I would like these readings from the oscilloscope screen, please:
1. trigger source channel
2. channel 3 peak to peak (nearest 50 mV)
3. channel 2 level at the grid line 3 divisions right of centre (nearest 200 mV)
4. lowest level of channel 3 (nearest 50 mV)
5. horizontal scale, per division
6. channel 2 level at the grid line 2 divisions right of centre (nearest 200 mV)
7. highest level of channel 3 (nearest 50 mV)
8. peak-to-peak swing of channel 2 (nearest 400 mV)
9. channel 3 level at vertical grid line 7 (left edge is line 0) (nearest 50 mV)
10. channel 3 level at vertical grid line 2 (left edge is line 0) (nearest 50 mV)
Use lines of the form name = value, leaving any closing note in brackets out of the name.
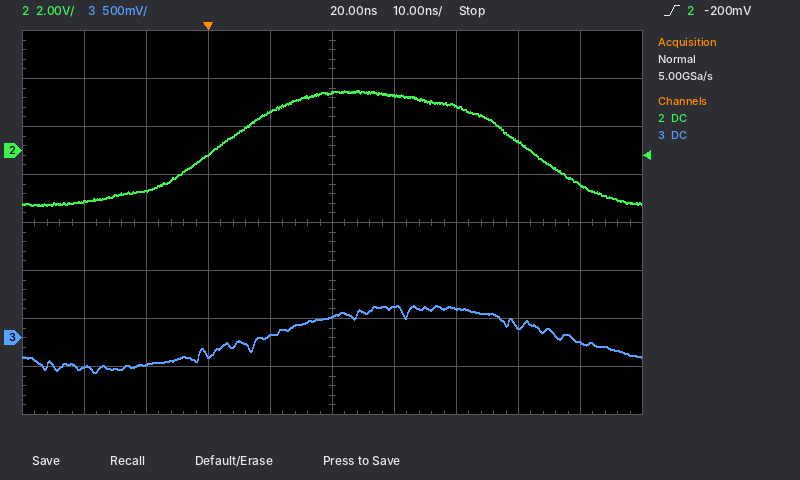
trigger source channel = channel 2
channel 3 peak to peak = 700 mV
channel 2 level at the grid line 3 divisions right of centre = 400 mV
lowest level of channel 3 = -350 mV
horizontal scale, per division = 10 ns
channel 2 level at the grid line 2 divisions right of centre = 1.8 V
highest level of channel 3 = 350 mV
peak-to-peak swing of channel 2 = 4.8 V
channel 3 level at vertical grid line 7 (left edge is line 0) = 300 mV
channel 3 level at vertical grid line 2 (left edge is line 0) = -300 mV
